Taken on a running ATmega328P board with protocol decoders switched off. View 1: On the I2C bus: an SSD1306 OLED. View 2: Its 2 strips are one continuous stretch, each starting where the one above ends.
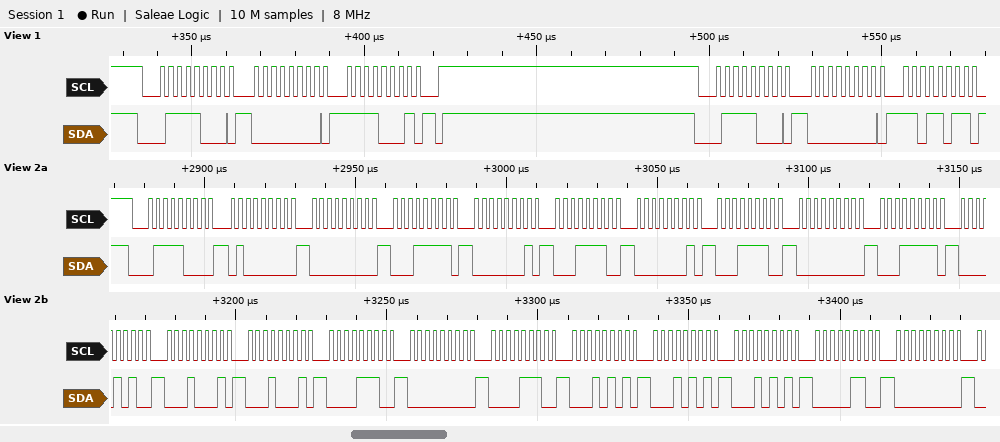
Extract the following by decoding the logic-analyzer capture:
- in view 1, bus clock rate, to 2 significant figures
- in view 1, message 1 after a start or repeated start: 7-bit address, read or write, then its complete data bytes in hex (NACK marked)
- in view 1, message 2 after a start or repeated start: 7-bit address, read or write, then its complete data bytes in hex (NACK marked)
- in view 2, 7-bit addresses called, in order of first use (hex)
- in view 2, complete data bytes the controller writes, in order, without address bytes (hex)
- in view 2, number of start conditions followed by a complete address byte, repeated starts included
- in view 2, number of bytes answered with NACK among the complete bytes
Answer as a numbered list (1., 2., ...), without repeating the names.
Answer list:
1. 400 kHz
2. 0x3C write: 00 F1
3. 0x3C write: 00 DB
4. 0x3C
5. 40 00 1F 01 1E 01 1E 00 1F 0A 11 11 0E 00 0E 15 15 15 06 00
6. 1
7. 0
